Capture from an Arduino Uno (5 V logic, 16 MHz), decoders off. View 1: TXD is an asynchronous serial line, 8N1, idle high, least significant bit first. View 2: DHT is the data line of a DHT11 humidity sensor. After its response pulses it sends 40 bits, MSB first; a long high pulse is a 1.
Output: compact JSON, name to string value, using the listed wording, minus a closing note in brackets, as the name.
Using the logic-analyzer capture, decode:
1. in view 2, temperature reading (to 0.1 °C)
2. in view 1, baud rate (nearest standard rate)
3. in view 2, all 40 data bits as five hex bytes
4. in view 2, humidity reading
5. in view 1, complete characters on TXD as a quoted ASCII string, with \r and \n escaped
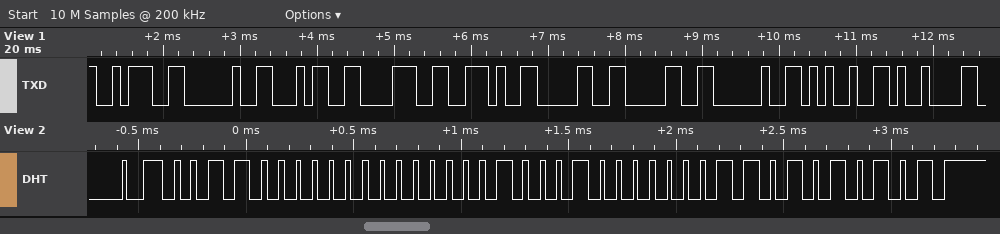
{"in view 2, temperature reading": "34.3 °C", "in view 1, baud rate": "9600 baud", "in view 2, all 40 data bits as five hex bytes": "30 00 22 03 55", "in view 2, humidity reading": "48 %", "in view 1, complete characters on TXD as a quoted ASCII string, with \\r and \\n escaped": "\": 48.00 %\\t\""}
